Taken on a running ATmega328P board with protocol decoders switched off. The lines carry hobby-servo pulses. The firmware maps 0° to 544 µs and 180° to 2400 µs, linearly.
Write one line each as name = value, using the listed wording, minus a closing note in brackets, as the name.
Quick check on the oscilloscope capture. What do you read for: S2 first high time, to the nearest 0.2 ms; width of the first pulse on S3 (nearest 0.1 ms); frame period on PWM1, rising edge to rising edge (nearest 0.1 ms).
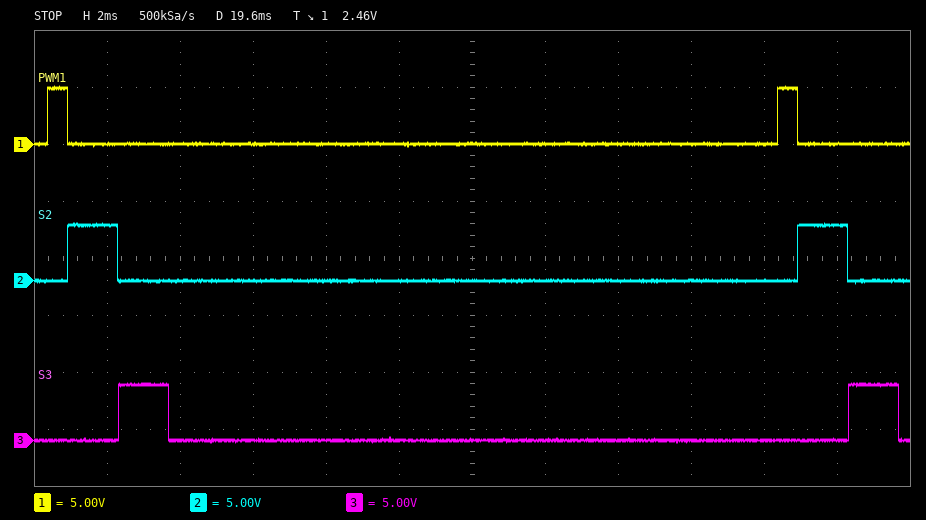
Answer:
S2 first high time, to the nearest 0.2 ms = 1.4 ms
width of the first pulse on S3 = 1.4 ms
frame period on PWM1, rising edge to rising edge = 20.0 ms
